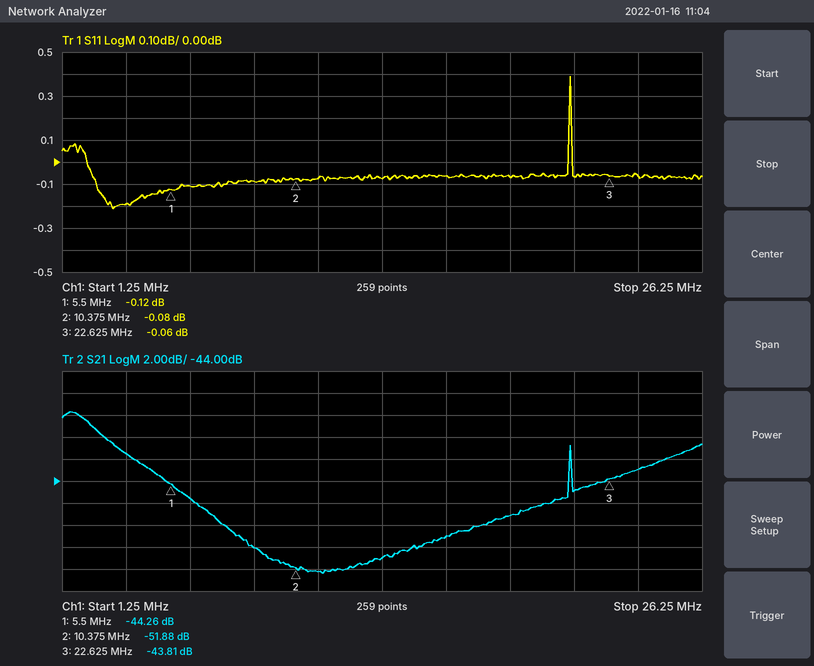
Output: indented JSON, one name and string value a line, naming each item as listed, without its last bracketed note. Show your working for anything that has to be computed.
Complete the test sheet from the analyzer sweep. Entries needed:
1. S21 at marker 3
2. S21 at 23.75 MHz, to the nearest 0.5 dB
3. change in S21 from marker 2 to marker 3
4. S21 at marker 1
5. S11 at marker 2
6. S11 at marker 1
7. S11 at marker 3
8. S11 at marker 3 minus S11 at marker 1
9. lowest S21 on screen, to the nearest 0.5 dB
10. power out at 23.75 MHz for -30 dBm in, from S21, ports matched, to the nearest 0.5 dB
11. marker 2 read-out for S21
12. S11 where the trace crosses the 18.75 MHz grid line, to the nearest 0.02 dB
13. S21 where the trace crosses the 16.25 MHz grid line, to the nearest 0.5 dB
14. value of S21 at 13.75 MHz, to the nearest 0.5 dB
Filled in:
{
  "S21 at marker 3": "-43.81 dB",
  "S21 at 23.75 MHz, to the nearest 0.5 dB": "-43.0 dB",
  "change in S21 from marker 2 to marker 3": "-43.81 − (-51.88) = 8.07 dB",
  "S21 at marker 1": "-44.26 dB",
  "S11 at marker 2": "-0.08 dB",
  "S11 at marker 1": "-0.12 dB",
  "S11 at marker 3": "-0.06 dB",
  "S11 at marker 3 minus S11 at marker 1": "-0.06 − (-0.12) = 0.06 dB",
  "lowest S21 on screen, to the nearest 0.5 dB": "-52.5 dB",
  "power out at 23.75 MHz for -30 dBm in, from S21, ports matched, to the nearest 0.5 dB": "-30 dBm + (-43.0 dB) = -73.0 dBm",
  "marker 2 read-out for S21": "-51.88 dB",
  "S11 where the trace crosses the 18.75 MHz grid line, to the nearest 0.02 dB": "-0.06 dB",
  "S21 where the trace crosses the 16.25 MHz grid line, to the nearest 0.5 dB": "-49.0 dB",
  "value of S21 at 13.75 MHz, to the nearest 0.5 dB": "-51.0 dB"
}
